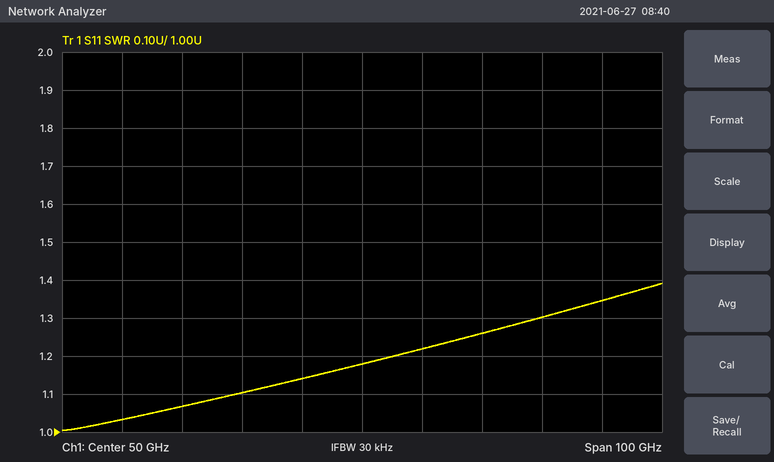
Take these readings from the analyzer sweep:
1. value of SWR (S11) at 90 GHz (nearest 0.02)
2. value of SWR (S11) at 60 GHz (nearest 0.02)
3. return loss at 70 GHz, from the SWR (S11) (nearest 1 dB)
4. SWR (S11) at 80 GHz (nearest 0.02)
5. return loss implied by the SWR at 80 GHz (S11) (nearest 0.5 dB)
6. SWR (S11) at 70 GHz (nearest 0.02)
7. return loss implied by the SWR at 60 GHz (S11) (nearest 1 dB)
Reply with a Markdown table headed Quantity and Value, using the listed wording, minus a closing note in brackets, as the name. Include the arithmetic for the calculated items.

| Quantity | Value |
|---|---|
| value of SWR (S11) at 90 GHz | 1.34 |
| value of SWR (S11) at 60 GHz | 1.22 |
| return loss at 70 GHz, from the SWR (S11) | −20 log10((1.26 − 1)/(1.26 + 1)) ≈ 19 dB |
| SWR (S11) at 80 GHz | 1.30 |
| return loss implied by the SWR at 80 GHz (S11) | −20 log10((1.3 − 1)/(1.3 + 1)) ≈ 17.7 dB, so 17.5 dB to the nearest 0.5 dB |
| SWR (S11) at 70 GHz | 1.26 |
| return loss implied by the SWR at 60 GHz (S11) | −20 log10((1.22 − 1)/(1.22 + 1)) ≈ 20 dB |
